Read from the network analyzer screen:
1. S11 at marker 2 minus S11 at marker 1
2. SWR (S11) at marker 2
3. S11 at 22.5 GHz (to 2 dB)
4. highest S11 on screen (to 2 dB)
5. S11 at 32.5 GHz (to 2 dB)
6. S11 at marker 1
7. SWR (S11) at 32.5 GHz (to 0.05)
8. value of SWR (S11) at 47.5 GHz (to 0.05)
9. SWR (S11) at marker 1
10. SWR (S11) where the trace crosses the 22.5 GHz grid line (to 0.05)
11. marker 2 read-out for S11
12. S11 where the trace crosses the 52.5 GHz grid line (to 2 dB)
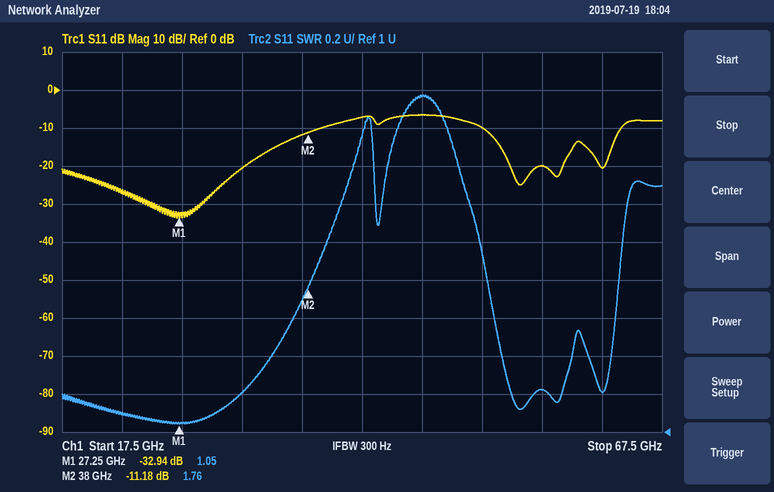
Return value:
21.76 dB
1.76
-26 dB
-6 dB
-20 dB
-32.94 dB
1.20
2.75
1.05
1.10
-11.18 dB
-10 dB
